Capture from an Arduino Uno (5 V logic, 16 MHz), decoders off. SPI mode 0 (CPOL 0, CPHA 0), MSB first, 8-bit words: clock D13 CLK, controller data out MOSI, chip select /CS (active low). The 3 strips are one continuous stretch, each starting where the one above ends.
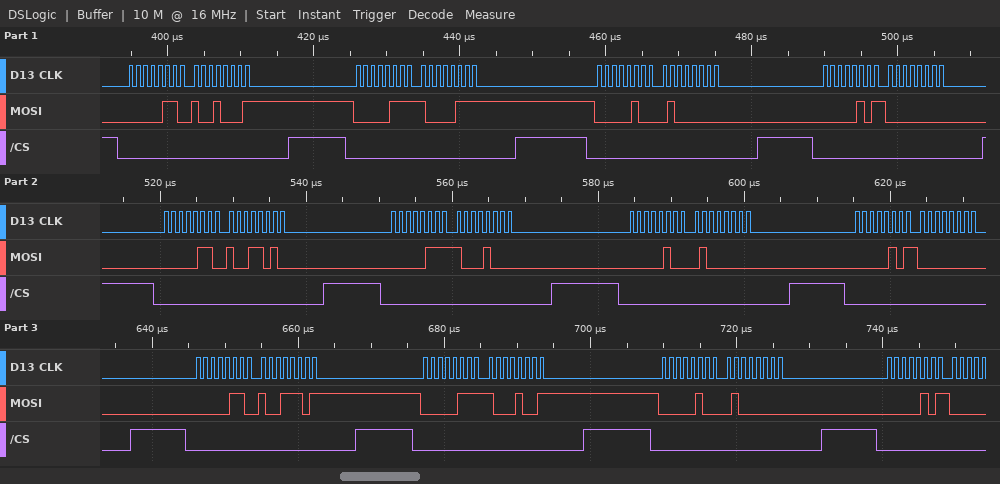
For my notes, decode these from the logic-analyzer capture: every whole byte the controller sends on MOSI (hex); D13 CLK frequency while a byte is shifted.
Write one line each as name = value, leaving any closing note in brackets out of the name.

every whole byte the controller sends on MOSI = 06 91 07 87 04 40 05 00 06 9A 07 88 04 40 05 00 06 9D 07 89 04 40 05
D13 CLK frequency while a byte is shifted = 1 MHz
